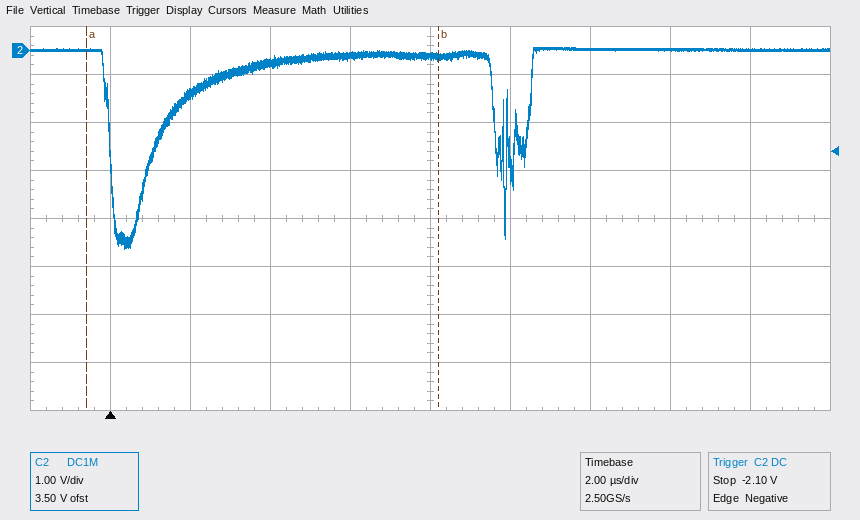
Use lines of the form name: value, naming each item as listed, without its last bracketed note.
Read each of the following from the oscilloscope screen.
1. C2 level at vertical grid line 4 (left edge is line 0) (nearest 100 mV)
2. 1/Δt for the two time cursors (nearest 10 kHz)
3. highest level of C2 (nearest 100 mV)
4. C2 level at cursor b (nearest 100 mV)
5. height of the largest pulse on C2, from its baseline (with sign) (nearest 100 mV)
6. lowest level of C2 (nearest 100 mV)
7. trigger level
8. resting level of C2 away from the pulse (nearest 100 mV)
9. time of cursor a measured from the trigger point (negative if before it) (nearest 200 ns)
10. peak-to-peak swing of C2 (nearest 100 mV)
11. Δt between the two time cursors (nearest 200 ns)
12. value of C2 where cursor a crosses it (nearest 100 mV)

C2 level at vertical grid line 4 (left edge is line 0): -100 mV
1/Δt for the two time cursors: 110 kHz
highest level of C2: 100 mV
C2 level at cursor b: -100 mV
height of the largest pulse on C2, from its baseline (with sign): -4.1 V
lowest level of C2: -4.1 V
trigger level: -2.10 V
resting level of C2 away from the pulse: 0.0 V
time of cursor a measured from the trigger point (negative if before it): -600 ns
peak-to-peak swing of C2: 4.2 V
Δt between the two time cursors: 8.8 µs
value of C2 where cursor a crosses it: 0.0 V
